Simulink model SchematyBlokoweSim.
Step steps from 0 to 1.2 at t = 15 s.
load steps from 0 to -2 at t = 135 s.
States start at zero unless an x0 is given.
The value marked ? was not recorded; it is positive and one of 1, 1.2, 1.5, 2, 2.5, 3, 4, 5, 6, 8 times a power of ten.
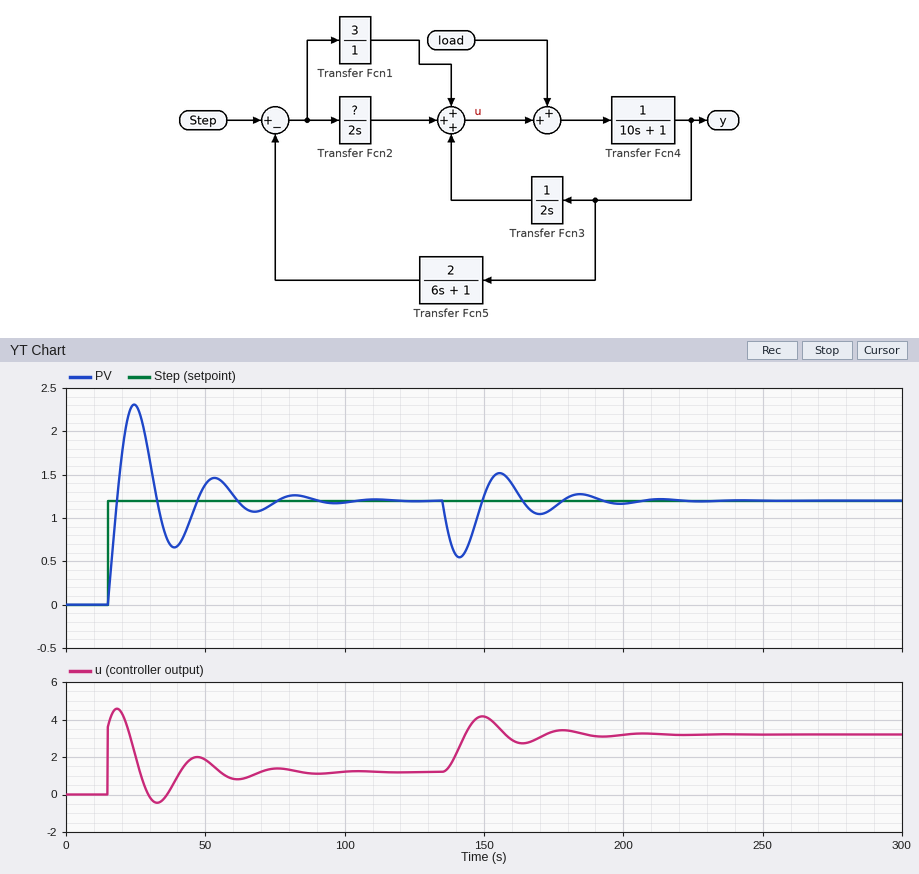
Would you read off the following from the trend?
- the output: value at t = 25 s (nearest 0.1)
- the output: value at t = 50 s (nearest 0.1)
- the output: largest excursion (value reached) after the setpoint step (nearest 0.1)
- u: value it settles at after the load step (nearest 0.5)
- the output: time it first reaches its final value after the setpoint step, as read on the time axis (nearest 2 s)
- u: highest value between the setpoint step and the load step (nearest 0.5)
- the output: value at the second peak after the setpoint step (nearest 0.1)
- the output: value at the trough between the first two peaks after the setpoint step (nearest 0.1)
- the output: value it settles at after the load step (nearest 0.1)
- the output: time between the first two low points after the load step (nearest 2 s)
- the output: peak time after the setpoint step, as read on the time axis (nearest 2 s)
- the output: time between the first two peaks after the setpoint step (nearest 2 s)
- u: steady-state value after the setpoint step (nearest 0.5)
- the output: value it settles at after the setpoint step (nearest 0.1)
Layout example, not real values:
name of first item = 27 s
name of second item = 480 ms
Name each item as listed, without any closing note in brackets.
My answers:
the output: value at t = 25 s = 2.3
the output: value at t = 50 s = 1.4
the output: largest excursion (value reached) after the setpoint step = 2.3
u: value it settles at after the load step = 3.0
the output: time it first reaches its final value after the setpoint step, as read on the time axis = 18 s
u: highest value between the setpoint step and the load step = 4.5
the output: value at the second peak after the setpoint step = 1.5
the output: value at the trough between the first two peaks after the setpoint step = 0.7
the output: value it settles at after the load step = 1.2
the output: time between the first two low points after the load step = 28 s
the output: peak time after the setpoint step, as read on the time axis = 24 s
the output: time between the first two peaks after the setpoint step = 28 s
u: steady-state value after the setpoint step = 1.0
the output: value it settles at after the setpoint step = 1.2
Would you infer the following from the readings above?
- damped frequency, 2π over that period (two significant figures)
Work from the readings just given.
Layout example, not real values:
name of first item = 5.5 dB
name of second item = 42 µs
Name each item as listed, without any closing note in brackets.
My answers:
damped frequency, 2π over that period = 0.22 rad/s
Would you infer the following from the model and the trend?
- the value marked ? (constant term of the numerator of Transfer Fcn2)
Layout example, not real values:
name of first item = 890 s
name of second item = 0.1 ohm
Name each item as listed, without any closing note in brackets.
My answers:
the value marked ? = 1
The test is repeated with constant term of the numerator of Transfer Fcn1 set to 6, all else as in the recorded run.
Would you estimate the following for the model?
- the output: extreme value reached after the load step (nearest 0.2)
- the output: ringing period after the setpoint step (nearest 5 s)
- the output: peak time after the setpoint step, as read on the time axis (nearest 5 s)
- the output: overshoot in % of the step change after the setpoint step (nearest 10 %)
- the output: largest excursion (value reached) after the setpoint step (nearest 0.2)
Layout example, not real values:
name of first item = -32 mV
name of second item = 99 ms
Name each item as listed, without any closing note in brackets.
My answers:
the output: extreme value reached after the load step = 0.8
the output: ringing period after the setpoint step = 15 s
the output: peak time after the setpoint step, as read on the time axis = 20 s
the output: overshoot in % of the step change after the setpoint step = 70 %
the output: largest excursion (value reached) after the setpoint step = 2.0
